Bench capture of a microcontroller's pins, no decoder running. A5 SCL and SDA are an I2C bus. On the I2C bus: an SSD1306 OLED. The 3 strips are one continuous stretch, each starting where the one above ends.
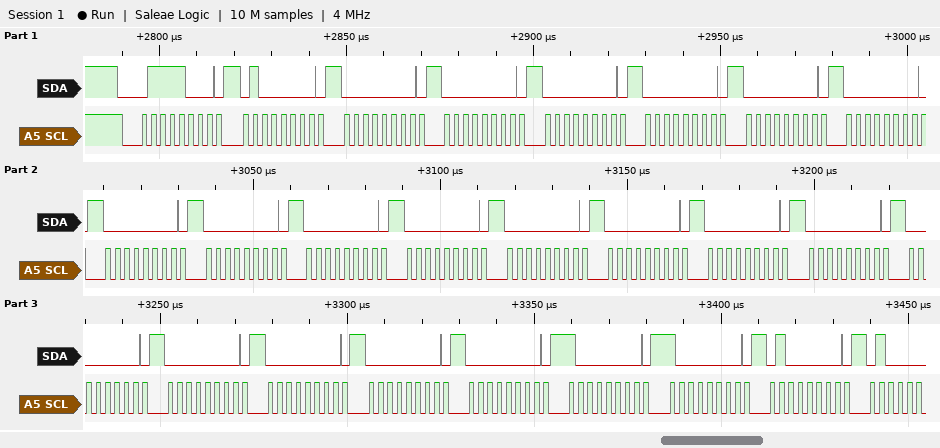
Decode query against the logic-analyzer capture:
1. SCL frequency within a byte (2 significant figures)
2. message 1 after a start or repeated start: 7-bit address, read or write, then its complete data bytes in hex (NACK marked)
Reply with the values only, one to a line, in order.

400 kHz
0x3C write: 40 00 00 00 00 00 00 00 00 00 00 00 00 00 00 00 00 00 00 00 80 80 40
